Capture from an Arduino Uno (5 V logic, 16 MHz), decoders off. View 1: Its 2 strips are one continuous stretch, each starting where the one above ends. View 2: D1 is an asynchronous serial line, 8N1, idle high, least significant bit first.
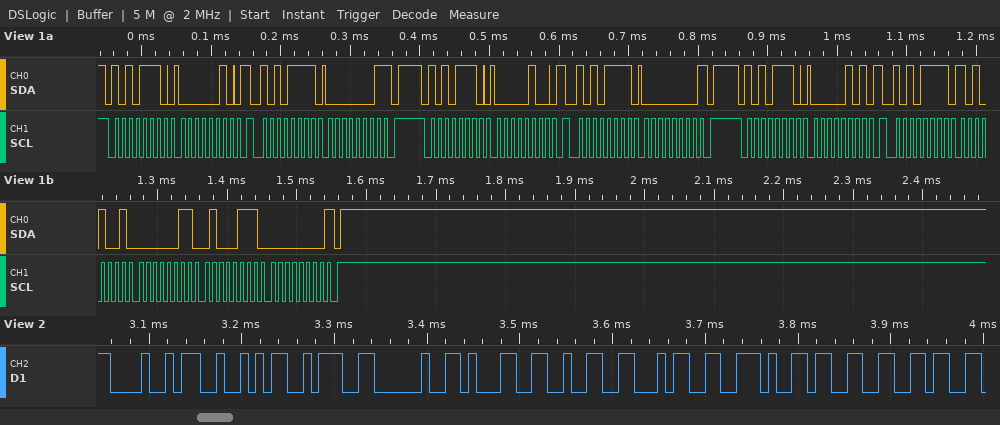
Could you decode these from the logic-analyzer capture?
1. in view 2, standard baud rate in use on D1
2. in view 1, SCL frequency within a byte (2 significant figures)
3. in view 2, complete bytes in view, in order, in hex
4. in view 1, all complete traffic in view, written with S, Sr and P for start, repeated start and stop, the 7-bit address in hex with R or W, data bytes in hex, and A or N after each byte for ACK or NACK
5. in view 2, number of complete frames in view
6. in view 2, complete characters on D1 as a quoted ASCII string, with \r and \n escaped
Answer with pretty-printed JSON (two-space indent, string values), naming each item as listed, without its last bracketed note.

{
  "in view 2, standard baud rate in use on D1": "115200 baud",
  "in view 1, SCL frequency within a byte": "100 kHz",
  "in view 2, complete bytes in view, in order, in hex": "0x48 0x52 0x3A 0x20 0x31 0x32 0x34 0x2E 0x33 0x36",
  "in view 1, all complete traffic in view, written with S, Sr and P for start, repeated start and stop, the 7-bit address in hex with R or W, data bytes in hex, and A or N after each byte for ACK or NACK": "S 57W A 02 A Sr 57R A 01 N P S 57W A 04 A Sr 57R A 00 N P S 57W A 05 A Sr 57R A A9 A 03 A 47 A 00 N P",
  "in view 2, number of complete frames in view": "10",
  "in view 2, complete characters on D1 as a quoted ASCII string, with \\r and \\n escaped": "\"HR: 124.36\""
}
